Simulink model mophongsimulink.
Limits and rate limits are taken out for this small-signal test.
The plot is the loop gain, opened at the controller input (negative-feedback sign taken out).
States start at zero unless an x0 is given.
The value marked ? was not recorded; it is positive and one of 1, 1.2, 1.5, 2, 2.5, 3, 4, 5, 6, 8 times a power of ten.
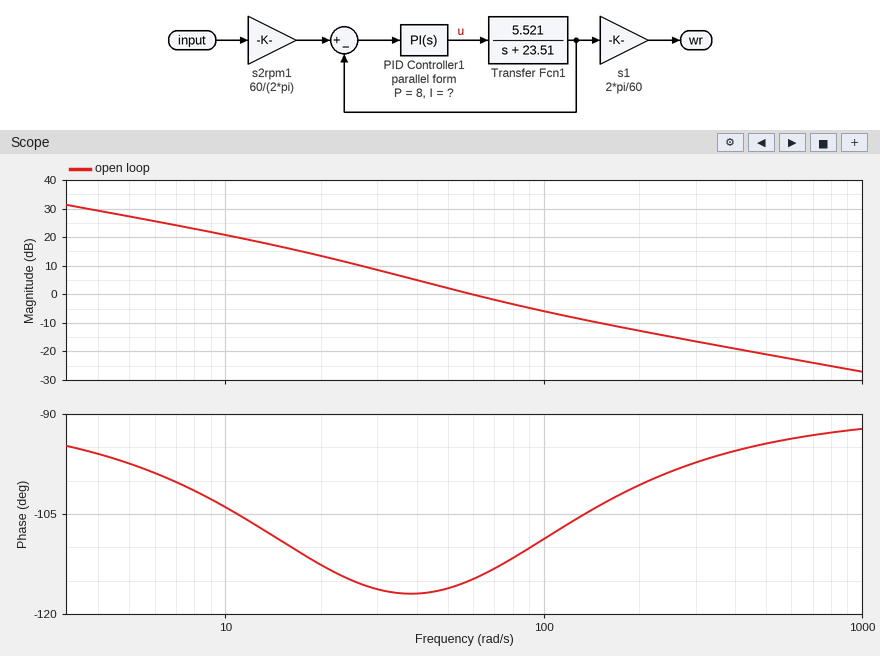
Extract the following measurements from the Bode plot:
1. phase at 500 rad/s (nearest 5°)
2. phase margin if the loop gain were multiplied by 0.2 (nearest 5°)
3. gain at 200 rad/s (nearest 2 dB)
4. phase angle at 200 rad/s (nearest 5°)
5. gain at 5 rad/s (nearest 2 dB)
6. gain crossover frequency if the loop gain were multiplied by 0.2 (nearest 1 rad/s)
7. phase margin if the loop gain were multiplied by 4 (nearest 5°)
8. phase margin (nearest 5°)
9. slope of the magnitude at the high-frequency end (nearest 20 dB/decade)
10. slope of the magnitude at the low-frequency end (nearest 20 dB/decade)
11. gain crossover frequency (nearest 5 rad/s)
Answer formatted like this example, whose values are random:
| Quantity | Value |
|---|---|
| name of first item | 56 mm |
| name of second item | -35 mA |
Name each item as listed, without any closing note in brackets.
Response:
| Quantity | Value |
|---|---|
| phase at 500 rad/s | -95° |
| phase margin if the loop gain were multiplied by 0.2 | 70° |
| gain at 200 rad/s | -12 dB |
| phase angle at 200 rad/s | -100° |
| gain at 5 rad/s | 28 dB |
| gain crossover frequency if the loop gain were multiplied by 0.2 | 19 rad/s |
| phase margin if the loop gain were multiplied by 4 | 80° |
| phase margin | 65° |
| slope of the magnitude at the high-frequency end | -20 dB/decade |
| slope of the magnitude at the low-frequency end | -20 dB/decade |
| gain crossover frequency | 60 rad/s |
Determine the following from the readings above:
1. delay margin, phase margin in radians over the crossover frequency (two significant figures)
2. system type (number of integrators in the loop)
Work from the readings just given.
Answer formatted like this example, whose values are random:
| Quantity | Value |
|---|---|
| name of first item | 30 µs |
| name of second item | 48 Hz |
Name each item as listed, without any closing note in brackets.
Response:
| Quantity | Value |
|---|---|
| delay margin, phase margin in radians over the crossover frequency | 0.019 s |
| system type | 1 |
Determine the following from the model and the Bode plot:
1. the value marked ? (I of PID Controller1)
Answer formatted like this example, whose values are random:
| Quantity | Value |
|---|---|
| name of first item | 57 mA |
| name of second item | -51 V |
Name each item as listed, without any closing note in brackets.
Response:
| Quantity | Value |
|---|---|
| the value marked ? | 500 |
